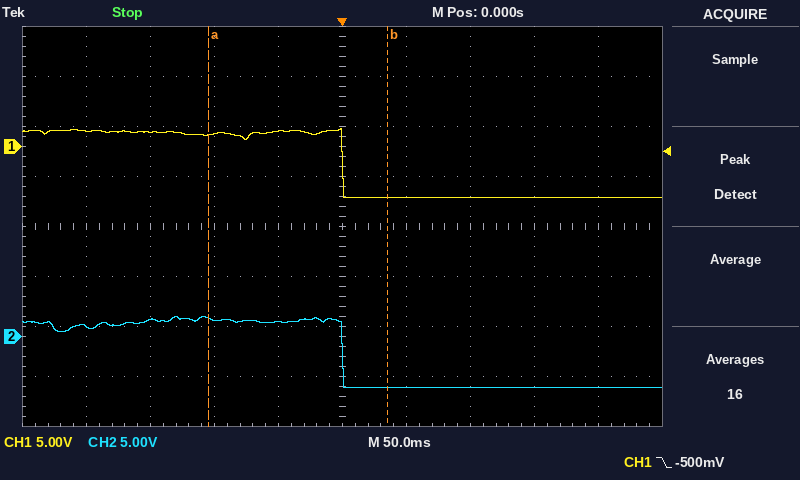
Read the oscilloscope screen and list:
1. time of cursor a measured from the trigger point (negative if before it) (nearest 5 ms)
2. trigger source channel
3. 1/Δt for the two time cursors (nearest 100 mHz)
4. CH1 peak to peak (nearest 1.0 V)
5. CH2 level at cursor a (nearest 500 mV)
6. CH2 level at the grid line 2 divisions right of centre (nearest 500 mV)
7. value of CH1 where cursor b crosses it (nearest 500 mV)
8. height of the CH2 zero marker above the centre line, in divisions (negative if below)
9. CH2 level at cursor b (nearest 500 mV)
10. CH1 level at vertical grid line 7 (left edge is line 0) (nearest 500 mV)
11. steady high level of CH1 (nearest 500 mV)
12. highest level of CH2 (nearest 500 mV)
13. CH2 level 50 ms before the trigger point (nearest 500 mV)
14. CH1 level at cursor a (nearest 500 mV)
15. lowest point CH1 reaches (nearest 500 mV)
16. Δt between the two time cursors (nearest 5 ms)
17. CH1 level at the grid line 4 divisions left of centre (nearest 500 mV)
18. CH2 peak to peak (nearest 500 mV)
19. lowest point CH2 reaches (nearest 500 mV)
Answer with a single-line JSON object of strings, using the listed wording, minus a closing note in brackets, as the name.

{"time of cursor a measured from the trigger point (negative if before it)": "-105 ms", "trigger source channel": "CH1", "1/Δt for the two time cursors": "7.1 Hz", "CH1 peak to peak": "7.0 V", "CH2 level at cursor a": "2.0 V", "CH2 level at the grid line 2 divisions right of centre": "-5.0 V", "value of CH1 where cursor b crosses it": "-5.0 V", "height of the CH2 zero marker above the centre line, in divisions": "-2.2 div", "CH2 level at cursor b": "-5.0 V", "CH1 level at vertical grid line 7 (left edge is line 0)": "-5.0 V", "steady high level of CH1": "1.5 V", "highest level of CH2": "2.0 V", "CH2 level 50 ms before the trigger point": "1.5 V", "CH1 level at cursor a": "1.0 V", "lowest point CH1 reaches": "-5.0 V", "Δt between the two time cursors": "140 ms", "CH1 level at the grid line 4 divisions left of centre": "1.5 V", "CH2 peak to peak": "7.0 V", "lowest point CH2 reaches": "-5.0 V"}
